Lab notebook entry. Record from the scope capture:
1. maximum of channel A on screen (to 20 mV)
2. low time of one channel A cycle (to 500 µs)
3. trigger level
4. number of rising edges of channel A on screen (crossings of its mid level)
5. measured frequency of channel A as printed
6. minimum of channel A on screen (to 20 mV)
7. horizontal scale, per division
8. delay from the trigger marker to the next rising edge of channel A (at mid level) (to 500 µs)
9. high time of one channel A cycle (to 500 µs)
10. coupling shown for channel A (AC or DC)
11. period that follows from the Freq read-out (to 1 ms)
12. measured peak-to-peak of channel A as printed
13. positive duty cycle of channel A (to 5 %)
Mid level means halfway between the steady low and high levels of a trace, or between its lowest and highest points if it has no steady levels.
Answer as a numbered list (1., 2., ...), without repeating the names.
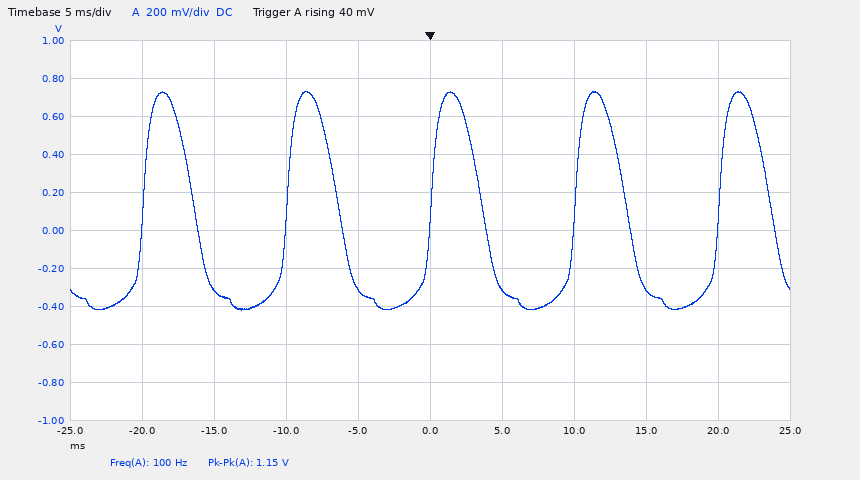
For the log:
1. 740 mV
2. 6.5 ms
3. 40 mV
4. 5
5. 100 Hz
6. -420 mV
7. 5 ms
8. 10.0 ms
9. 3.5 ms
10. DC
11. 10 ms
12. 1.15 V
13. 35 %
